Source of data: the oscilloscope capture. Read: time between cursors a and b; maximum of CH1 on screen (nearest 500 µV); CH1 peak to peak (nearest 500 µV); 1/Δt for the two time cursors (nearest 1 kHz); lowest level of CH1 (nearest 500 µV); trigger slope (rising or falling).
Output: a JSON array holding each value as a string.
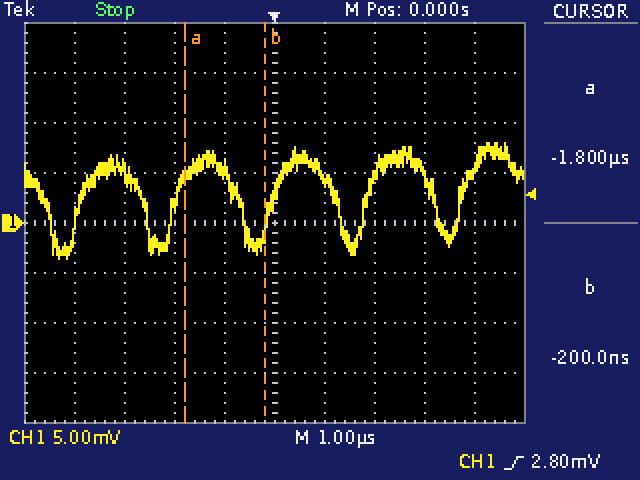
["1.6 µs", "8.0 mV", "11.5 mV", "625 kHz", "-3.5 mV", "rising"]
